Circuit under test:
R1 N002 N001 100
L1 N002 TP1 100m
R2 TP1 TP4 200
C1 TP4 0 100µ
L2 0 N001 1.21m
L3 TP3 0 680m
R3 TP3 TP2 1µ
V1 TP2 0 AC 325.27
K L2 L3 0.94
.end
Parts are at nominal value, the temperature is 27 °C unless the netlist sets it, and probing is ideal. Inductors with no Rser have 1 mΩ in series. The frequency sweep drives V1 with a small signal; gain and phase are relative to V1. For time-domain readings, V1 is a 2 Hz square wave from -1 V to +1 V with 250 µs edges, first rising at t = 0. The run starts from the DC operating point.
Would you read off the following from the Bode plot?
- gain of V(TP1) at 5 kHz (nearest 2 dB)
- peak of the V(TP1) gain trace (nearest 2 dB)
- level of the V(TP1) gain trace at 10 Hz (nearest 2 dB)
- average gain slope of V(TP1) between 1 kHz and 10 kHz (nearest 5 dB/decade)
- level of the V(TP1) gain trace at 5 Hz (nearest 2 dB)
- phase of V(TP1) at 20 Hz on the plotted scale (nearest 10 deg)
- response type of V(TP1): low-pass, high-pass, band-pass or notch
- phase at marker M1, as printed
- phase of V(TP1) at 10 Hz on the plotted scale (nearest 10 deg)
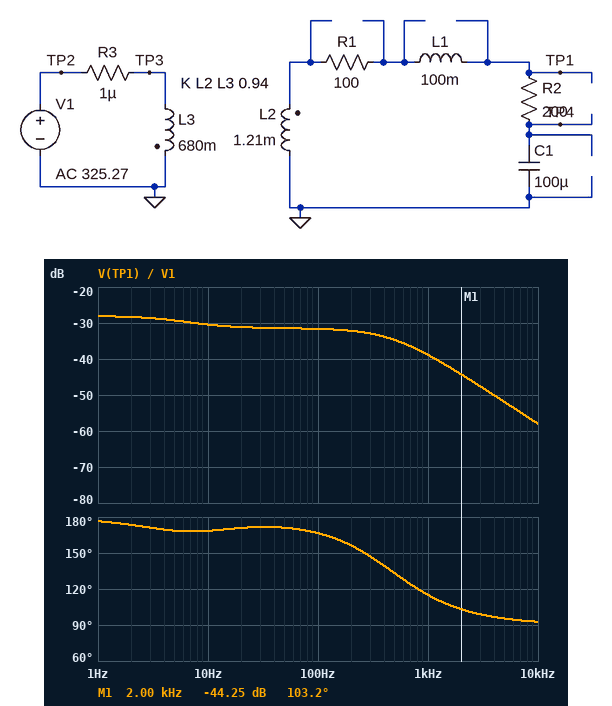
-52 dB
-28 dB
-30 dB
-20 dB/decade
-30 dB
170 deg
low-pass
103.2 deg
170 deg
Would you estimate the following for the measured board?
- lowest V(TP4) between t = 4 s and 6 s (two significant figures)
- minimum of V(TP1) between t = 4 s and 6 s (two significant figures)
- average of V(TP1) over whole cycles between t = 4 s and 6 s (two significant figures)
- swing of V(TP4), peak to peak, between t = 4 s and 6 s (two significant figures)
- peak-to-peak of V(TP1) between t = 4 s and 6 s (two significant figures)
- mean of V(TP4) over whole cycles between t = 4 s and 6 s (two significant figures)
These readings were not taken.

-79 mV
-79 mV
-39 mV
79 mV
79 mV
-39 mV
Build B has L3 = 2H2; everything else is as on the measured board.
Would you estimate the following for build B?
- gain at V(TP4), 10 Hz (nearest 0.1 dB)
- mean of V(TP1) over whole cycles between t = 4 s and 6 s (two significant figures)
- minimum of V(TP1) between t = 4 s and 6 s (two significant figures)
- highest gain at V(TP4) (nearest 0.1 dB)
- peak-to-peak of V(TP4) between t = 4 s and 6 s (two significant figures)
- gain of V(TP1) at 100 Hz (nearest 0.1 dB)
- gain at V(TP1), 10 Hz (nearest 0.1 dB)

-39.6 dB
-22 mV
-44 mV
-33.1 dB
44 mV
-36.7 dB
-35.5 dB
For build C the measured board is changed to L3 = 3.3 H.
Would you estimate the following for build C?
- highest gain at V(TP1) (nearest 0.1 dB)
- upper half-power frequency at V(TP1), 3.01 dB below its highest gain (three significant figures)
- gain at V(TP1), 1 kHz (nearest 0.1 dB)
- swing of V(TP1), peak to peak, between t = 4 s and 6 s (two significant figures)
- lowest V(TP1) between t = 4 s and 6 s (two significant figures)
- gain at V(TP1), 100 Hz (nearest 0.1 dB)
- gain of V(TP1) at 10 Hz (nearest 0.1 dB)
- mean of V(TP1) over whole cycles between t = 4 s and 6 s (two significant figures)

-34.9 dB
17.7 Hz
-45.7 dB
36 mV
-36 mV
-38.5 dB
-37.3 dB
-18 mV
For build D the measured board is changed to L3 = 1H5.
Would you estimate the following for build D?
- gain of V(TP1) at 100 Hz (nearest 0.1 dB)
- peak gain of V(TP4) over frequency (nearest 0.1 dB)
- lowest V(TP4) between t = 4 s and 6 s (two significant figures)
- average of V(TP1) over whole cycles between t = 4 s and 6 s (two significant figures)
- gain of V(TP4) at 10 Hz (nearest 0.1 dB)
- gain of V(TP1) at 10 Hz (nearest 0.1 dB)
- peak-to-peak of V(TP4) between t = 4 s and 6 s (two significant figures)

-35.1 dB
-31.5 dB
-53 mV
-27 mV
-38.0 dB
-33.9 dB
53 mV
